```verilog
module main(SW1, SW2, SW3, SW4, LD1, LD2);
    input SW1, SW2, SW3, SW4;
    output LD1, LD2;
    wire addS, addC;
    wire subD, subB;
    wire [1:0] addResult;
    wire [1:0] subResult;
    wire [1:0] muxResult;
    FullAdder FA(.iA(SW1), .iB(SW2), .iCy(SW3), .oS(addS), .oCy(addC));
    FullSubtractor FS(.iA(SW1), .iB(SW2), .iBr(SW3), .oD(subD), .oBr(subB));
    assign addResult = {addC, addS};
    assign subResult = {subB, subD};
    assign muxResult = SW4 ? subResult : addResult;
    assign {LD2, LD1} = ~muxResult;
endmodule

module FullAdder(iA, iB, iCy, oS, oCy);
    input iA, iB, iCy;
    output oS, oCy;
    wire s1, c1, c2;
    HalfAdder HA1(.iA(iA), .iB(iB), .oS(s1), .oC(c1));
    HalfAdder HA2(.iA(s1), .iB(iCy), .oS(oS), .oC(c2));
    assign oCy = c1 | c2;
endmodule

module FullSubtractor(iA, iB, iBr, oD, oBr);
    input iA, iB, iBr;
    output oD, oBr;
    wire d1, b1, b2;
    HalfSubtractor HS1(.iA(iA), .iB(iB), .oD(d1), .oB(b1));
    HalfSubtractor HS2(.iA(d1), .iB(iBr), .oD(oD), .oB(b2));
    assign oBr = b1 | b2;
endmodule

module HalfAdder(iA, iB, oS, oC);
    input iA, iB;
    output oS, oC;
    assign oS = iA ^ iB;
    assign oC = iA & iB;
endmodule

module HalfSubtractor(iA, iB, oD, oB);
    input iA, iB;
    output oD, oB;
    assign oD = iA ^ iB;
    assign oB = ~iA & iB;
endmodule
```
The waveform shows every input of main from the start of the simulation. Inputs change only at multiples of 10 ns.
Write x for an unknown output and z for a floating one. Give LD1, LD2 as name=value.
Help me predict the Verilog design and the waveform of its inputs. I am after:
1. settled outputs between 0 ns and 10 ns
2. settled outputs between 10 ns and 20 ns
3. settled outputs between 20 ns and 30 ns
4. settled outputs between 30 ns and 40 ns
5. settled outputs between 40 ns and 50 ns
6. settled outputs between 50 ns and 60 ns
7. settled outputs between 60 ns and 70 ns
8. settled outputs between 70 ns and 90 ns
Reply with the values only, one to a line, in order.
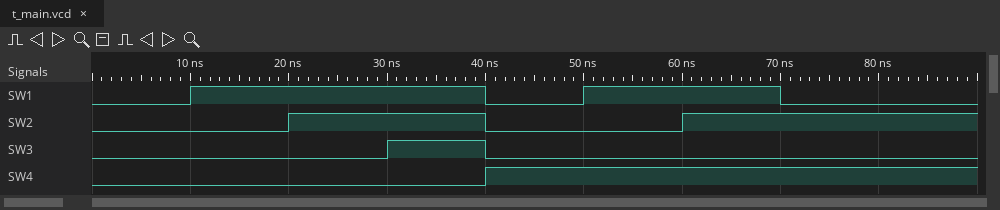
LD1=1, LD2=1
LD1=0, LD2=1
LD1=1, LD2=0
LD1=0, LD2=0
LD1=1, LD2=1
LD1=0, LD2=1
LD1=1, LD2=1
LD1=0, LD2=0
